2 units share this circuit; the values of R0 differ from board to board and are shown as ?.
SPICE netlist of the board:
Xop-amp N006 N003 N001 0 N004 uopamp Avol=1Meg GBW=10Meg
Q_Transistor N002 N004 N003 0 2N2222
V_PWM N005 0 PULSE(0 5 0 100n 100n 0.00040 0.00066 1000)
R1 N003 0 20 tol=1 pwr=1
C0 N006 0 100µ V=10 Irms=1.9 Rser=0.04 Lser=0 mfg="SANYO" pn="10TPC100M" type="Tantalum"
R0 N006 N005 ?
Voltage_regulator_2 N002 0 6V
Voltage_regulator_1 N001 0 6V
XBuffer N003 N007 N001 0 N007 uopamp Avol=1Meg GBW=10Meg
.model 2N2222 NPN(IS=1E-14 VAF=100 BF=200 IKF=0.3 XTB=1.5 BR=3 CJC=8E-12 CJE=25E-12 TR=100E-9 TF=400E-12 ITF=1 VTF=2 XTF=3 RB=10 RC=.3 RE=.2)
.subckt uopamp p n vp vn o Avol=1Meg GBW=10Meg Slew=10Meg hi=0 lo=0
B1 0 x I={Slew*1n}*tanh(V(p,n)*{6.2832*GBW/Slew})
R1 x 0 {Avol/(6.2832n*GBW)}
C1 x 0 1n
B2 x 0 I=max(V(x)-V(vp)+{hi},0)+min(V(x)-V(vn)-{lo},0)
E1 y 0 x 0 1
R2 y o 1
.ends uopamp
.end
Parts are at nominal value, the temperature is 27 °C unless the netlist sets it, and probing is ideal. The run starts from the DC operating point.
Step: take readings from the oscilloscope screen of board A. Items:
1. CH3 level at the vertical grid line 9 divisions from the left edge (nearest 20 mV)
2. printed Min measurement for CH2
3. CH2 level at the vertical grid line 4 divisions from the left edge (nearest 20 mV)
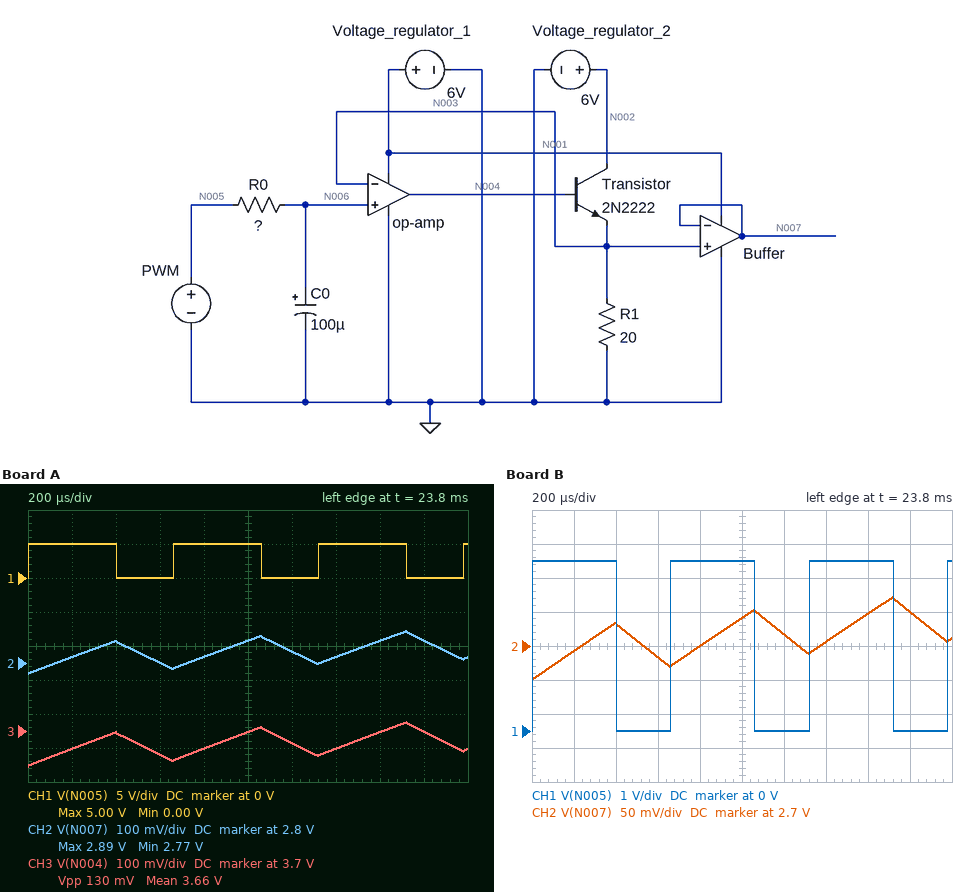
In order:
3.70 V
2.77 V
2.82 V
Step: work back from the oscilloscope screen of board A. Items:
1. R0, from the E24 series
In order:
91 Ω
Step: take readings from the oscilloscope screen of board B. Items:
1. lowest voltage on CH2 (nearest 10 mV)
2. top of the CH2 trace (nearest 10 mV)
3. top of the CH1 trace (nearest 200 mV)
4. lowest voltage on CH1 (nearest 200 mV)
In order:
2.65 V
2.77 V
5.0 V
0 V
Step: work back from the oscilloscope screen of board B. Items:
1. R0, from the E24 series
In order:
110 Ω
